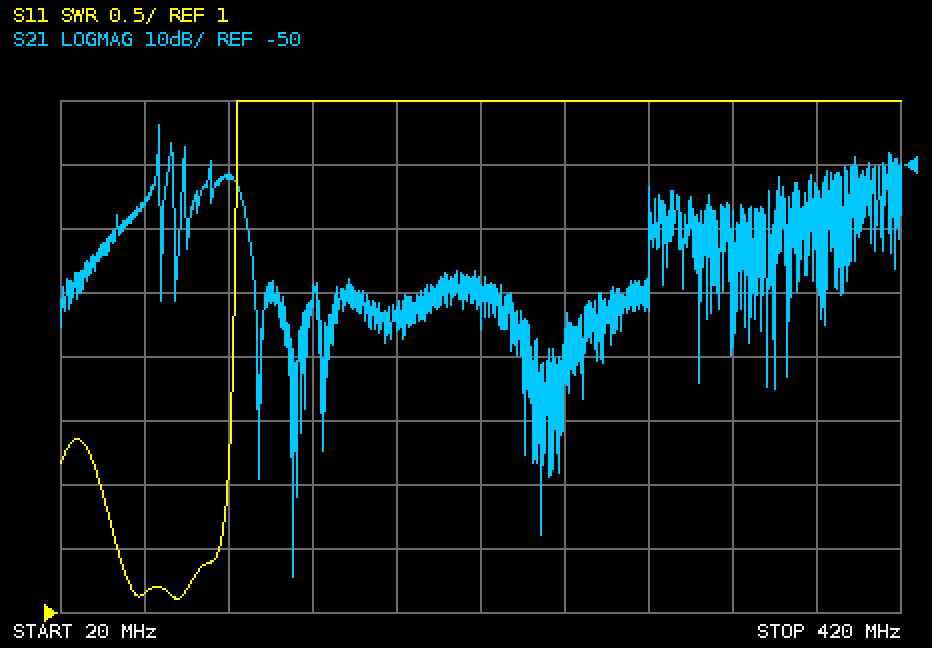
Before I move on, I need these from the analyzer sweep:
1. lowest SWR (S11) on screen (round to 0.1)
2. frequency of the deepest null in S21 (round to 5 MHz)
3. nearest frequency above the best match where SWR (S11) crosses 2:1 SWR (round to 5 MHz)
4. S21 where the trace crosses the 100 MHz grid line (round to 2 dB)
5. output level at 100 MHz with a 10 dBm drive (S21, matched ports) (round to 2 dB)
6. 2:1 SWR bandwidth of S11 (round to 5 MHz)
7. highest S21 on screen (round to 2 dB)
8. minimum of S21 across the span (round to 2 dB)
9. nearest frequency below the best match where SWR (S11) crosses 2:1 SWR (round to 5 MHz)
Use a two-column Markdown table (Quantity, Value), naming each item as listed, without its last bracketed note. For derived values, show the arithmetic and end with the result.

| Quantity | Value |
|---|---|
| lowest SWR (S11) on screen | 1.1 |
| frequency of the deepest null in S21 | 130 MHz |
| nearest frequency above the best match where SWR (S11) crosses 2:1 SWR | 100 MHz |
| S21 where the trace crosses the 100 MHz grid line | -52 dB |
| output level at 100 MHz with a 10 dBm drive (S21, matched ports) | 10 dBm + (-52 dB) = -42 dBm |
| 2:1 SWR bandwidth of S11 | 100 MHz − 40 MHz = 60 MHz |
| highest S21 on screen | -44 dB |
| minimum of S21 across the span | -114 dB |
| nearest frequency below the best match where SWR (S11) crosses 2:1 SWR | 40 MHz |
